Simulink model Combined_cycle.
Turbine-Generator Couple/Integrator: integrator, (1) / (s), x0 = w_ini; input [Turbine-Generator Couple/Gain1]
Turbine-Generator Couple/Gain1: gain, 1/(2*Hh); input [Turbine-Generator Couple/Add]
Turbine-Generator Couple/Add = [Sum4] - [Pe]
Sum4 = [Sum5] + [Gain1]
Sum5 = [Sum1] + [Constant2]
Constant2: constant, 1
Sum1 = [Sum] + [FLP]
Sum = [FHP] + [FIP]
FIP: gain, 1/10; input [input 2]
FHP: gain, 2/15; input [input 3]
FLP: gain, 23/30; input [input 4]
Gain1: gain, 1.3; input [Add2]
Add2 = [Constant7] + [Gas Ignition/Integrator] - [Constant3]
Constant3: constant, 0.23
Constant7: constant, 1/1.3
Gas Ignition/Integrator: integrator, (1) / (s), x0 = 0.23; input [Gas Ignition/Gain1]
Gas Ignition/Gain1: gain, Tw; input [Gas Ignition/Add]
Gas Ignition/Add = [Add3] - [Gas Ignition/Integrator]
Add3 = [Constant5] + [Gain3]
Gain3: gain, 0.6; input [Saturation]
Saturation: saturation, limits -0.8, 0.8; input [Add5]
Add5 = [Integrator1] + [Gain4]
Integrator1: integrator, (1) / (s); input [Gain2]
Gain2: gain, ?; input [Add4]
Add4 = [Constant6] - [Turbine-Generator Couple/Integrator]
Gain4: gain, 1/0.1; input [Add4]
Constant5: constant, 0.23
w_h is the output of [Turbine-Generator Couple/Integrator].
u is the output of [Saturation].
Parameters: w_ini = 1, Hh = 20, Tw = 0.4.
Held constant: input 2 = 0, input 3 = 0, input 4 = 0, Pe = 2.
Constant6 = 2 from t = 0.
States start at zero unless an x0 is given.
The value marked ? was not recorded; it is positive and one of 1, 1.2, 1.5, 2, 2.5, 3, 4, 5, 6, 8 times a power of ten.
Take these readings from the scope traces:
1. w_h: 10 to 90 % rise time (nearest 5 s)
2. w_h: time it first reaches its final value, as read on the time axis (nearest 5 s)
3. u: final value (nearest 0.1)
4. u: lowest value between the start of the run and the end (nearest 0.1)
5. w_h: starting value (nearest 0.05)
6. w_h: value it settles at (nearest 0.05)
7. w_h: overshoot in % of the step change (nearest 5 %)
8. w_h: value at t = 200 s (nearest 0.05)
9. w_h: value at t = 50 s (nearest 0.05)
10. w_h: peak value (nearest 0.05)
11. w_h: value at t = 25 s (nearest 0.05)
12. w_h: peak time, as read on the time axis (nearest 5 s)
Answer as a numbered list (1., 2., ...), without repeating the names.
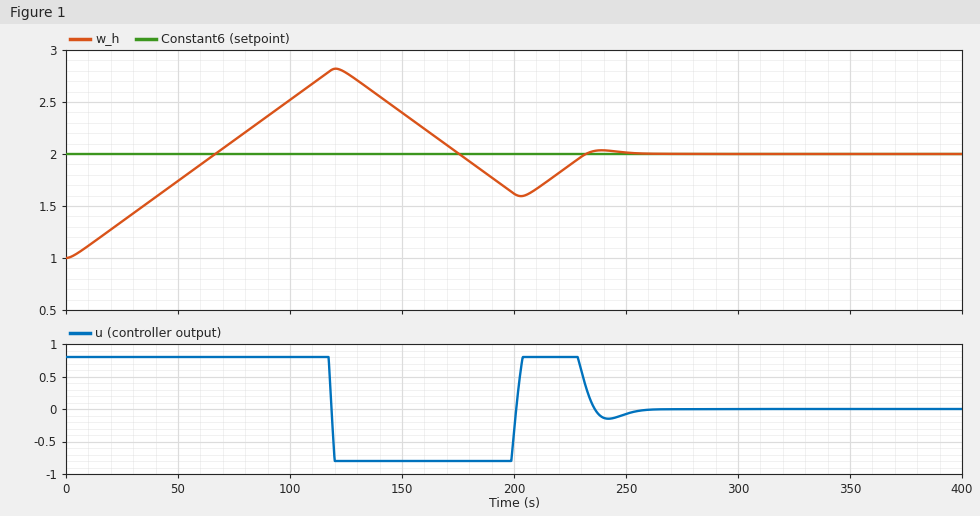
1. 50 s
2. 65 s
3. 0.0
4. -0.8
5. 1.00
6. 2.00
7. 80 %
8. 1.60
9. 1.75
10. 2.80
11. 1.35
12. 120 s
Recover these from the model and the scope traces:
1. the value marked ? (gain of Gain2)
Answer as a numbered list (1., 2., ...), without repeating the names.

1. 0.6
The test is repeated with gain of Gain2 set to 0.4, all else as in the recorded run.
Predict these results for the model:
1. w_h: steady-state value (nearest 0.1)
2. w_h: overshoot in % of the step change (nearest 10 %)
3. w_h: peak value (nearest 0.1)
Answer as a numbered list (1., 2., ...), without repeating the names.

1. 2.0
2. 70 %
3. 2.7
